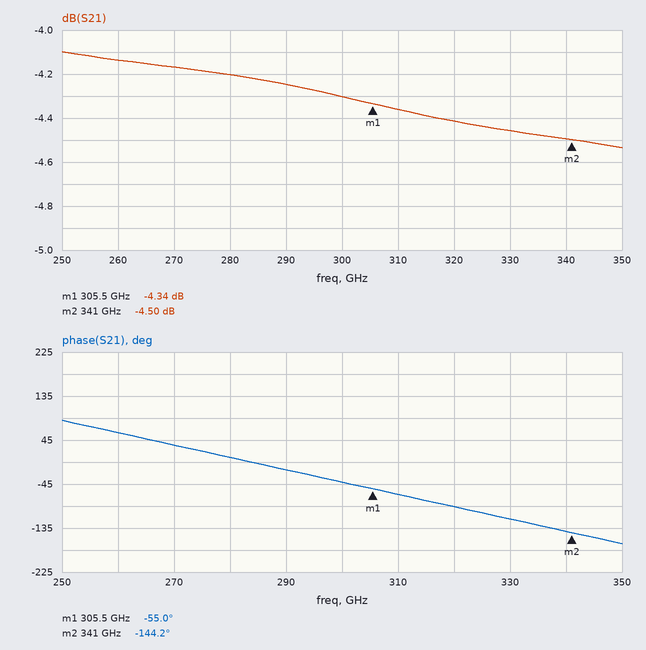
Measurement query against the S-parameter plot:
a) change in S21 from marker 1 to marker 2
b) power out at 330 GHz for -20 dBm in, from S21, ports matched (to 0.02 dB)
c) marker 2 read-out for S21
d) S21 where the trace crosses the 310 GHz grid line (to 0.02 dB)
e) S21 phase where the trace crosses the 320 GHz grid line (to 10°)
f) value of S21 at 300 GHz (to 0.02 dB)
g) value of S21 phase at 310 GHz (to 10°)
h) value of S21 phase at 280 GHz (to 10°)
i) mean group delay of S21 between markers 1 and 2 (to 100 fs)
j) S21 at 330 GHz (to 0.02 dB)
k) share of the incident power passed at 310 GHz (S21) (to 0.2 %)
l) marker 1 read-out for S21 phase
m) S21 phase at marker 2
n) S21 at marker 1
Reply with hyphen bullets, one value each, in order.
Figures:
- -0.16 dB
- -24.46 dBm
- -4.50 dB
- -4.36 dB
- -90°
- -4.30 dB
- -70°
- 10°
- 7.0 ps
- -4.46 dB
- 36.6 %
- -55.0°
- -144.2°
- -4.34 dB
